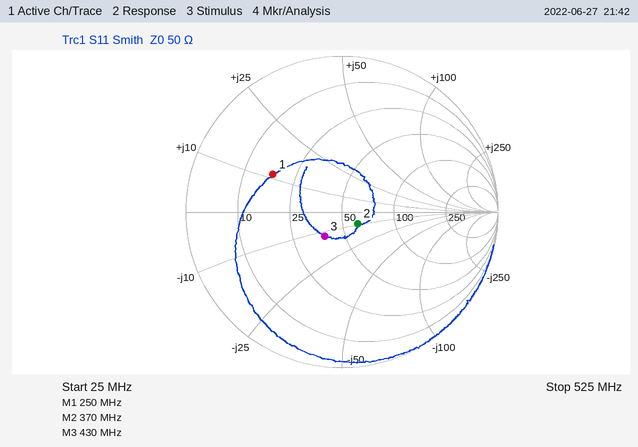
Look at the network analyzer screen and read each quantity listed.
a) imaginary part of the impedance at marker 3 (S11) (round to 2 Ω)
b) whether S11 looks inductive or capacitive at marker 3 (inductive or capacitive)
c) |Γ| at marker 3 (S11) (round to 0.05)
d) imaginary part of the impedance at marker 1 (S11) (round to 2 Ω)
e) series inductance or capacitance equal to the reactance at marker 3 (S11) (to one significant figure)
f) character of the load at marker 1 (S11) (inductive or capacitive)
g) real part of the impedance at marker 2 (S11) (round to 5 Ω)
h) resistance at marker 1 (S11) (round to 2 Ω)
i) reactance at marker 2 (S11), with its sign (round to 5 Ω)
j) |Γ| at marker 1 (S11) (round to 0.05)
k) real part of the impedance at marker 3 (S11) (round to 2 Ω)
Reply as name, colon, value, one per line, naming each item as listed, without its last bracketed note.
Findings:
imaginary part of the impedance at marker 3 (S11): -12 Ω
whether S11 looks inductive or capacitive at marker 3: capacitive
|Γ| at marker 3 (S11): 0.20
imaginary part of the impedance at marker 1 (S11): +12 Ω
series inductance or capacitance equal to the reactance at marker 3 (S11): 30 pF
character of the load at marker 1 (S11): inductive
real part of the impedance at marker 2 (S11): 60 Ω
resistance at marker 1 (S11): 18 Ω
reactance at marker 2 (S11), with its sign: -10 Ω
|Γ| at marker 1 (S11): 0.50
real part of the impedance at marker 3 (S11): 38 Ω
